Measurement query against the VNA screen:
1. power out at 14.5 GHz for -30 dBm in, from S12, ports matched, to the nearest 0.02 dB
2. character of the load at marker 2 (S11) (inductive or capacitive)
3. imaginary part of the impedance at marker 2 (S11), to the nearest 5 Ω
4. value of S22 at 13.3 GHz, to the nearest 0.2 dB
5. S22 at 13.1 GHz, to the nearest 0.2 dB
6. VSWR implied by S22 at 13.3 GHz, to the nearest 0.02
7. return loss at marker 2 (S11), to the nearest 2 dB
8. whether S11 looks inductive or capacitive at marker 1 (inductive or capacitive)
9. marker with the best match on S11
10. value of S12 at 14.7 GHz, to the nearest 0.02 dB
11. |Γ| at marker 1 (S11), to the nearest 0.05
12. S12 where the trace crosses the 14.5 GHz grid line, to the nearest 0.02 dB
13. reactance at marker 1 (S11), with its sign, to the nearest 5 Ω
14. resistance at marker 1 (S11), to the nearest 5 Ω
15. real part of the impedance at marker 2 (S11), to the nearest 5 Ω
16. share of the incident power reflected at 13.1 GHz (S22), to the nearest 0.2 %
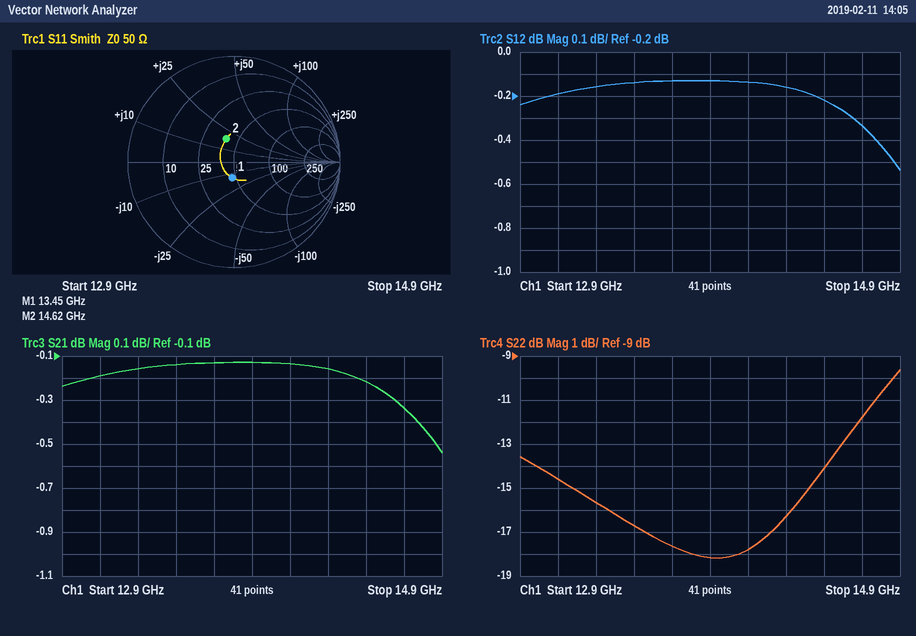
-30.22 dBm
inductive
+20 Ω
-15.6 dB
-14.6 dB
1.40
12 dB
capacitive
marker 1
-0.34 dB
0.15
-0.22 dB
-15 Ω
45 Ω
40 Ω
3.4 %
